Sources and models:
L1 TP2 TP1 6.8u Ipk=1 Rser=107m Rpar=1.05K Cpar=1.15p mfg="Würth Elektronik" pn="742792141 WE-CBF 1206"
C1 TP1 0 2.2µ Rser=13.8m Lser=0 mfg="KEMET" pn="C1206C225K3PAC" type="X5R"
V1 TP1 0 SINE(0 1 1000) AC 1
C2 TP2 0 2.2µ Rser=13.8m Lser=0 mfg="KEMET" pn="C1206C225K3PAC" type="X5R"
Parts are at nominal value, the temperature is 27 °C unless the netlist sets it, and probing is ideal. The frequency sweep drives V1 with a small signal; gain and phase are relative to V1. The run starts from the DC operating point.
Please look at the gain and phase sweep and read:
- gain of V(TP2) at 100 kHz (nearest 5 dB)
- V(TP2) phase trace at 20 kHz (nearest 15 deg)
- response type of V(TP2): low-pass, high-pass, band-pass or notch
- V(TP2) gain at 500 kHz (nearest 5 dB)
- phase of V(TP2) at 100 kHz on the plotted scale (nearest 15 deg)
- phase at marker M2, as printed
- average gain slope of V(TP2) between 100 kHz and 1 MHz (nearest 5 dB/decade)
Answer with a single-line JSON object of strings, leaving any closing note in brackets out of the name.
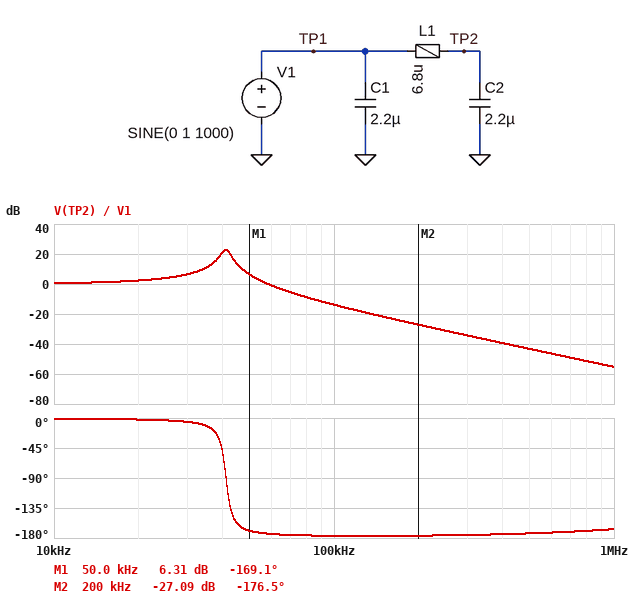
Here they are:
{"gain of V(TP2) at 100 kHz": "-15 dB", "V(TP2) phase trace at 20 kHz": "0 deg", "response type of V(TP2): low-pass, high-pass, band-pass or notch": "low-pass", "V(TP2) gain at 500 kHz": "-45 dB", "phase of V(TP2) at 100 kHz on the plotted scale": "-180 deg", "phase at marker M2, as printed": "-176.5 deg", "average gain slope of V(TP2) between 100 kHz and 1 MHz": "-40 dB/decade"}
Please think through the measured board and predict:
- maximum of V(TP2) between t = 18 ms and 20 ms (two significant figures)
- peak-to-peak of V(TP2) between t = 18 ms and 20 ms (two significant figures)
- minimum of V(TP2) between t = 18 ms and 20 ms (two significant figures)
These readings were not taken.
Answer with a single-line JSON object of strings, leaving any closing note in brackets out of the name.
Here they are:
{"maximum of V(TP2) between t = 18 ms and 20 ms": "1.0 V", "peak-to-peak of V(TP2) between t = 18 ms and 20 ms": "2.0 V", "minimum of V(TP2) between t = 18 ms and 20 ms": "-1.0 V"}
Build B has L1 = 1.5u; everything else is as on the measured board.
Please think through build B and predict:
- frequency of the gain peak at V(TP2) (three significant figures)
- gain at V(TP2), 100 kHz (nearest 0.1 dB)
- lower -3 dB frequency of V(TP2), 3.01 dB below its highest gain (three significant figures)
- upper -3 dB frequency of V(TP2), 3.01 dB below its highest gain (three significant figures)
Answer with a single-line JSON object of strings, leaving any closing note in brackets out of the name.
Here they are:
{"frequency of the gain peak at V(TP2)": "87.1 kHz", "gain at V(TP2), 100 kHz": "9.2 dB", "lower -3 dB frequency of V(TP2), 3.01 dB below its highest gain": "80.4 kHz", "upper -3 dB frequency of V(TP2), 3.01 dB below its highest gain": "93.4 kHz"}
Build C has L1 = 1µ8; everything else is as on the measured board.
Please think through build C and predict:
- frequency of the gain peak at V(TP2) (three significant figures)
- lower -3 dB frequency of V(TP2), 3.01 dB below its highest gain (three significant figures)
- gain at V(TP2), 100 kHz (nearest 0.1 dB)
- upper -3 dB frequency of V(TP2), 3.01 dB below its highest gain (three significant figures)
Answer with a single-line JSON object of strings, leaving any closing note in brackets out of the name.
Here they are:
{"frequency of the gain peak at V(TP2)": "79.6 kHz", "lower -3 dB frequency of V(TP2), 3.01 dB below its highest gain": "74.0 kHz", "gain at V(TP2), 100 kHz": "4.6 dB", "upper -3 dB frequency of V(TP2), 3.01 dB below its highest gain": "84.8 kHz"}
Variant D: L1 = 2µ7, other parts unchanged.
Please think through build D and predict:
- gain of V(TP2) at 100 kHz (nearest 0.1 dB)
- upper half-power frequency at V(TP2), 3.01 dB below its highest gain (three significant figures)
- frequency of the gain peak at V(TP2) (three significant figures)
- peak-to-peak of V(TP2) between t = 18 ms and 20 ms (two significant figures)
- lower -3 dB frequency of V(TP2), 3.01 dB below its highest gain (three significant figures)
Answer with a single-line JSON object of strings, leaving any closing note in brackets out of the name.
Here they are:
{"gain of V(TP2) at 100 kHz": "-2.6 dB", "upper half-power frequency at V(TP2), 3.01 dB below its highest gain": "68.6 kHz", "frequency of the gain peak at V(TP2)": "65.1 kHz", "peak-to-peak of V(TP2) between t = 18 ms and 20 ms": "2.0 V", "lower -3 dB frequency of V(TP2), 3.01 dB below its highest gain": "61.4 kHz"}
